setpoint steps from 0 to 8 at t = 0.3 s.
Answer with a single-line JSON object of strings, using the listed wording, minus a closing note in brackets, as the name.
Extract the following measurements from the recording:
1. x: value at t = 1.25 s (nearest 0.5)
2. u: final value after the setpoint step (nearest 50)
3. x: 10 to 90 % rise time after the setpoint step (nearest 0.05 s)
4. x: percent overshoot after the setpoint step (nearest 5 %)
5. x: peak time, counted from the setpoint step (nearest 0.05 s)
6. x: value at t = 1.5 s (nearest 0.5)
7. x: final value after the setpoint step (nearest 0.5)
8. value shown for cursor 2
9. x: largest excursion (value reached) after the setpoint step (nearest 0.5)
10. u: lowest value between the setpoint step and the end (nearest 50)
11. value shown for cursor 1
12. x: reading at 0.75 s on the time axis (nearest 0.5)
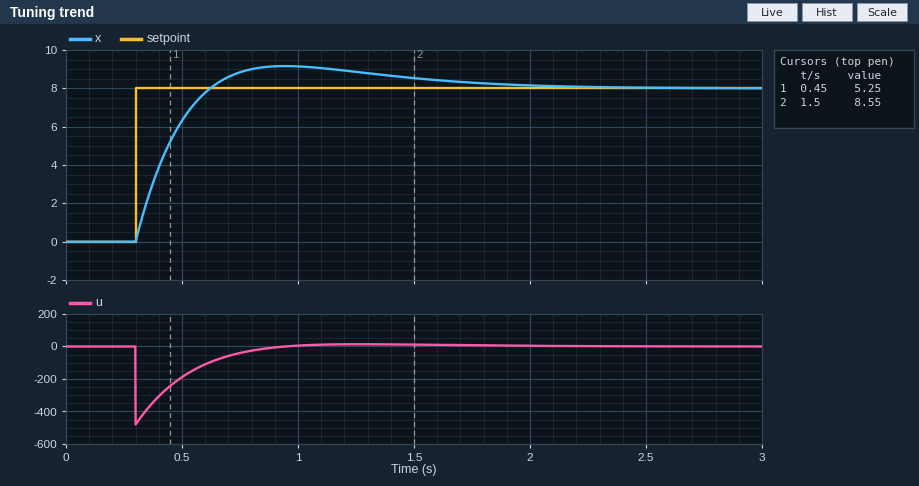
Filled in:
{"x: value at t = 1.25 s": "9.0", "u: final value after the setpoint step": "0", "x: 10 to 90 % rise time after the setpoint step": "0.25 s", "x: percent overshoot after the setpoint step": "15 %", "x: peak time, counted from the setpoint step": "0.65 s", "x: value at t = 1.5 s": "8.5", "x: final value after the setpoint step": "8.0", "value shown for cursor 2": "8.55", "x: largest excursion (value reached) after the setpoint step": "9.0", "u: lowest value between the setpoint step and the end": "-500", "value shown for cursor 1": "5.25", "x: reading at 0.75 s on the time axis": "9.0"}
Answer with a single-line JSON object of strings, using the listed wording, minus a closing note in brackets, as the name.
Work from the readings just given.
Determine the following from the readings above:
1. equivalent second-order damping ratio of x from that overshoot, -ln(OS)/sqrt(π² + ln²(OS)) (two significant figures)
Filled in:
{"equivalent second-order damping ratio of x from that overshoot, -ln(OS)/sqrt(π² + ln²(OS))": "0.52"}
